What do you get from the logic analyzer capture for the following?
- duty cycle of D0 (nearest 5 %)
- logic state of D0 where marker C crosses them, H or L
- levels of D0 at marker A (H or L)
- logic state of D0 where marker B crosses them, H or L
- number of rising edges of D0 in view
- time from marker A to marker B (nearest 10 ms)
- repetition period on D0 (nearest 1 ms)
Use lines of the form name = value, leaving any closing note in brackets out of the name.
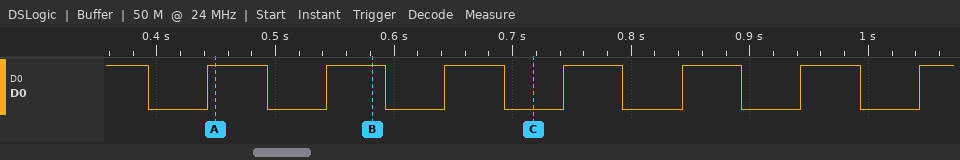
duty cycle of D0 = 50 %
logic state of D0 where marker C crosses them, H or L = D0=L
levels of D0 at marker A = D0=H
logic state of D0 where marker B crosses them, H or L = D0=H
number of rising edges of D0 in view = 7
time from marker A to marker B = 130 ms
repetition period on D0 = 100 ms
